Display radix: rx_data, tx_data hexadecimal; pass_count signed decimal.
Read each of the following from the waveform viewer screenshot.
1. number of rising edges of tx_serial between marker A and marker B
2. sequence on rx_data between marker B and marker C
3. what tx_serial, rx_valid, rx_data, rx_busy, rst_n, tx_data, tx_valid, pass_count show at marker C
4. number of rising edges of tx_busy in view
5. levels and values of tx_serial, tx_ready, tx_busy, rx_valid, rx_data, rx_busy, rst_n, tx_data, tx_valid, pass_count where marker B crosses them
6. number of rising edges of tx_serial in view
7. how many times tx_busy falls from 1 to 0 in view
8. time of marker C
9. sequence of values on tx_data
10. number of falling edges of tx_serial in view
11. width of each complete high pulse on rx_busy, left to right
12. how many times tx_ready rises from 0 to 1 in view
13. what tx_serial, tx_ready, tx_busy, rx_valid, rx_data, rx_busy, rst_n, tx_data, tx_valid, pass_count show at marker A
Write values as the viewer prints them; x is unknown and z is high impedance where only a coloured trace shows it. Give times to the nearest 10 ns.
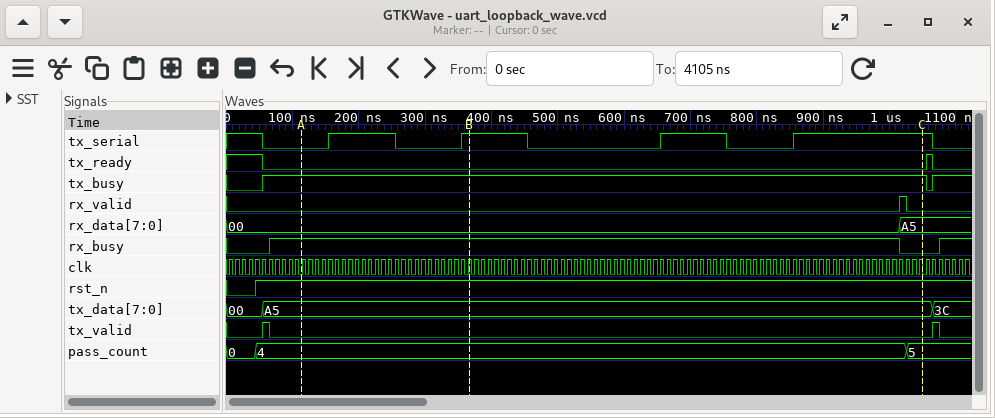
2
00, A5
tx_serial=1, rx_valid=0, rx_data=A5, rx_busy=0, rst_n=1, tx_data=A5, tx_valid=0, pass_count=5
2
tx_serial=1, tx_ready=0, tx_busy=1, rx_valid=0, rx_data=00, rx_busy=1, rst_n=1, tx_data=A5, tx_valid=0, pass_count=4
4
1
1050 ns
00, A5, 3C
5
950 ns
1
tx_serial=0, tx_ready=0, tx_busy=1, rx_valid=0, rx_data=00, rx_busy=1, rst_n=1, tx_data=A5, tx_valid=0, pass_count=4
